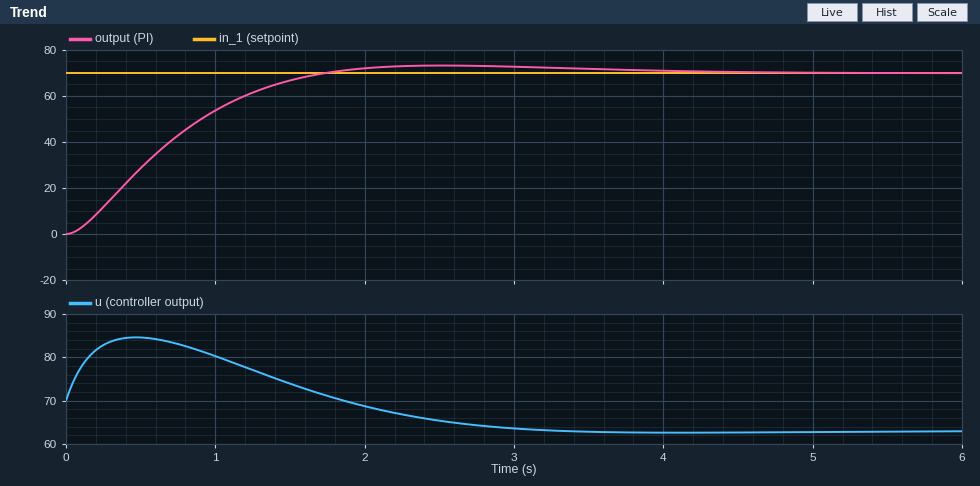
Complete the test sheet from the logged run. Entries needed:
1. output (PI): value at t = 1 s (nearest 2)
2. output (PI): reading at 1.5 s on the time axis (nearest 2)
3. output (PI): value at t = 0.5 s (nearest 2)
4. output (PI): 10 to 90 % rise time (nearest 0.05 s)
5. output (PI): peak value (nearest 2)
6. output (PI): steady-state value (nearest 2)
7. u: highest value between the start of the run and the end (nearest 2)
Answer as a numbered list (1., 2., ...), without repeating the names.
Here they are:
1. 54
2. 66
3. 28
4. 1.15 s
5. 74
6. 70
7. 84
